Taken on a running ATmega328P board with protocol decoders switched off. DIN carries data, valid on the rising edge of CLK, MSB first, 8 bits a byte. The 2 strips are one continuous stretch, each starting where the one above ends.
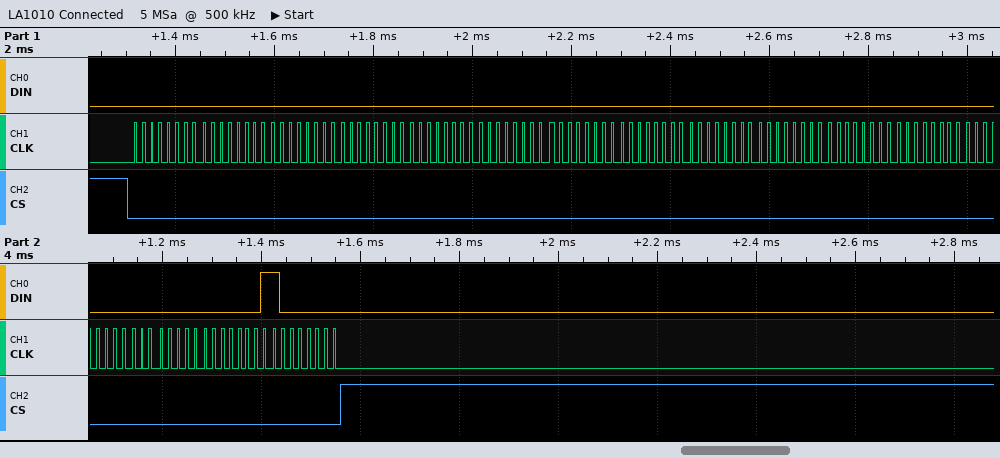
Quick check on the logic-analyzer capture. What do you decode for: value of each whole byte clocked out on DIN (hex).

0x00 0x00 0x00 0x00 0x00 0x00 0x00 0x00 0x00 0x00 0x00 0x00 0x00 0x00 0x01 0x80
